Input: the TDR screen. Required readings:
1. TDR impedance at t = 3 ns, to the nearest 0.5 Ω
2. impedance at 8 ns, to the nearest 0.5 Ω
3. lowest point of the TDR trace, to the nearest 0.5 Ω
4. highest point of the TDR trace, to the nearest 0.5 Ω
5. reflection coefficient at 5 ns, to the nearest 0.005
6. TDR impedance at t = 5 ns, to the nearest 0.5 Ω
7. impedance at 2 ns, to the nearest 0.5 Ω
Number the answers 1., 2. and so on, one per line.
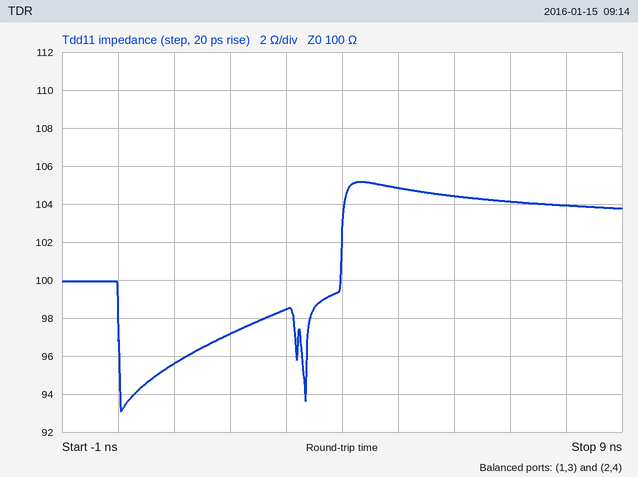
1. 98.5 Ω
2. 104.0 Ω
3. 93.0 Ω
4. 105.0 Ω
5. +0.025
6. 105.0 Ω
7. 97.0 Ω
